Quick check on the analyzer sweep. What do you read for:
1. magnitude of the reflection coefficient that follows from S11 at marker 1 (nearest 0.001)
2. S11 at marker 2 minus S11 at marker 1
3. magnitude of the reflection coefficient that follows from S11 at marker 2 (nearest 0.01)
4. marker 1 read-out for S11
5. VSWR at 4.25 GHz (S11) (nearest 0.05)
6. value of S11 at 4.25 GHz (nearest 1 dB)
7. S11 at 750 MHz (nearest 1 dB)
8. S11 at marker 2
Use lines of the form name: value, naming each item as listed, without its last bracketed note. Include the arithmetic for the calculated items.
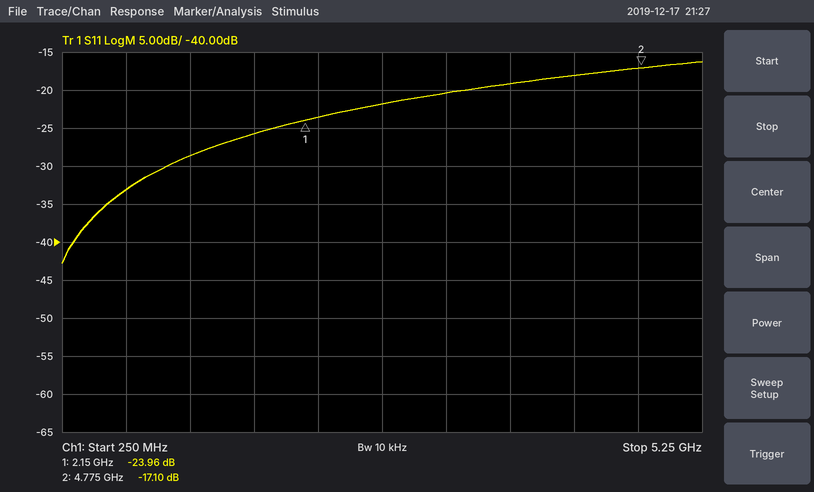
magnitude of the reflection coefficient that follows from S11 at marker 1: 10^(-23.96/20) ≈ 0.063
S11 at marker 2 minus S11 at marker 1: -17.1 − (-23.96) = 6.86 dB
magnitude of the reflection coefficient that follows from S11 at marker 2: 10^(-17.1/20) ≈ 0.14
marker 1 read-out for S11: -23.96 dB
VSWR at 4.25 GHz (S11): |Γ| = 10^(-18/20) = 0.1259; VSWR = (1 + 0.1259)/(1 − 0.1259) ≈ 1.29, so 1.30 to the nearest 0.05
value of S11 at 4.25 GHz: -18 dB
S11 at 750 MHz: -33 dB
S11 at marker 2: -17.10 dB
